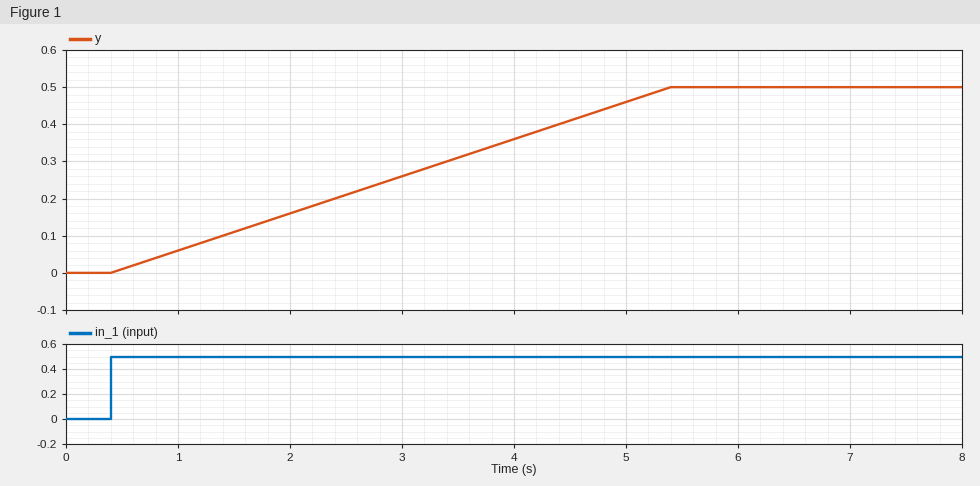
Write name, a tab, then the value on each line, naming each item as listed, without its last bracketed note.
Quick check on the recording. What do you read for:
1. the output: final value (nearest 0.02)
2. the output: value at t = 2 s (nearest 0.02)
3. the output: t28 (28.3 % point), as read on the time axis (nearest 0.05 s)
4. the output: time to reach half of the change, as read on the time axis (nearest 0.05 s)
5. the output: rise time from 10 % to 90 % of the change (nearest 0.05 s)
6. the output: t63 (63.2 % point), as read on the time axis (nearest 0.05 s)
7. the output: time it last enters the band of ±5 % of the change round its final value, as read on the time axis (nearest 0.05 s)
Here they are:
the output: final value	0.50
the output: value at t = 2 s	0.16
the output: t28 (28.3 % point), as read on the time axis	1.80 s
the output: time to reach half of the change, as read on the time axis	2.90 s
the output: rise time from 10 % to 90 % of the change	4.00 s
the output: t63 (63.2 % point), as read on the time axis	3.55 s
the output: time it last enters the band of ±5 % of the change round its final value, as read on the time axis	5.15 s
